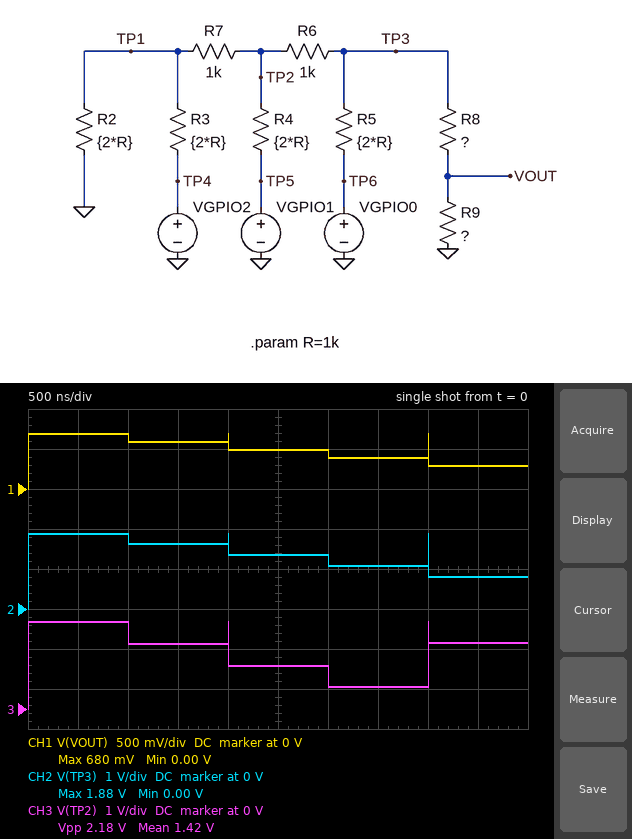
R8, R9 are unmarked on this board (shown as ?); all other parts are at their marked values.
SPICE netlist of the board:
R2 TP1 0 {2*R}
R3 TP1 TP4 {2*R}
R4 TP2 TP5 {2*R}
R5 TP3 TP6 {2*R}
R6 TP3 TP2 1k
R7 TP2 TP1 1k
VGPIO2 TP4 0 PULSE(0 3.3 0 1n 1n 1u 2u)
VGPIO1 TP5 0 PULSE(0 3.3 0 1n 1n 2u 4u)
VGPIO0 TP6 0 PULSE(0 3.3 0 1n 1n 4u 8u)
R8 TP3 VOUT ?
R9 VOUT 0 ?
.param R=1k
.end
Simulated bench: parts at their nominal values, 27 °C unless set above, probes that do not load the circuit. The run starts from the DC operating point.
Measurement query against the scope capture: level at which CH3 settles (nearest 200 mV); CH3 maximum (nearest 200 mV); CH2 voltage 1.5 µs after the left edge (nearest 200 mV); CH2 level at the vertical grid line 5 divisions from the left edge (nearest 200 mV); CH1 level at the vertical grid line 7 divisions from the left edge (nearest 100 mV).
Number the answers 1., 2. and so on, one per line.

1. 1.6 V
2. 2.2 V
3. 1.6 V
4. 1.4 V
5. 400 mV
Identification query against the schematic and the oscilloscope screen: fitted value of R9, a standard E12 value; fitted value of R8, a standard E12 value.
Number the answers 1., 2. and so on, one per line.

1. 680 Ω
2. 1.2 kΩ
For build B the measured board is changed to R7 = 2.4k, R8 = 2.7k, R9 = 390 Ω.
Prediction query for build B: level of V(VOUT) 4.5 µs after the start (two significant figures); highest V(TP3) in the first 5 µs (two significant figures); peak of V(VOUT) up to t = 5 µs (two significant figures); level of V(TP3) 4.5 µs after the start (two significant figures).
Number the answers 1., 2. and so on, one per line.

1. 120 mV
2. 2.2 V
3. 280 mV
4. 940 mV
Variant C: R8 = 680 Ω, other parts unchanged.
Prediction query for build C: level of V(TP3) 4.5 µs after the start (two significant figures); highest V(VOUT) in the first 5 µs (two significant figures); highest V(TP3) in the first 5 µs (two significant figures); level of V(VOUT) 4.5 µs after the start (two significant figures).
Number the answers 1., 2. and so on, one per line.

1. 710 mV
2. 830 mV
3. 1.7 V
4. 360 mV
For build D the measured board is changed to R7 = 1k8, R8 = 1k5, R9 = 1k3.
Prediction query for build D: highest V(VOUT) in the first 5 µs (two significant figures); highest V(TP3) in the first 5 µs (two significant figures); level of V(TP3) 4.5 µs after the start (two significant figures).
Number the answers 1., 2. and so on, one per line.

1. 1.0 V
2. 2.2 V
3. 910 mV
